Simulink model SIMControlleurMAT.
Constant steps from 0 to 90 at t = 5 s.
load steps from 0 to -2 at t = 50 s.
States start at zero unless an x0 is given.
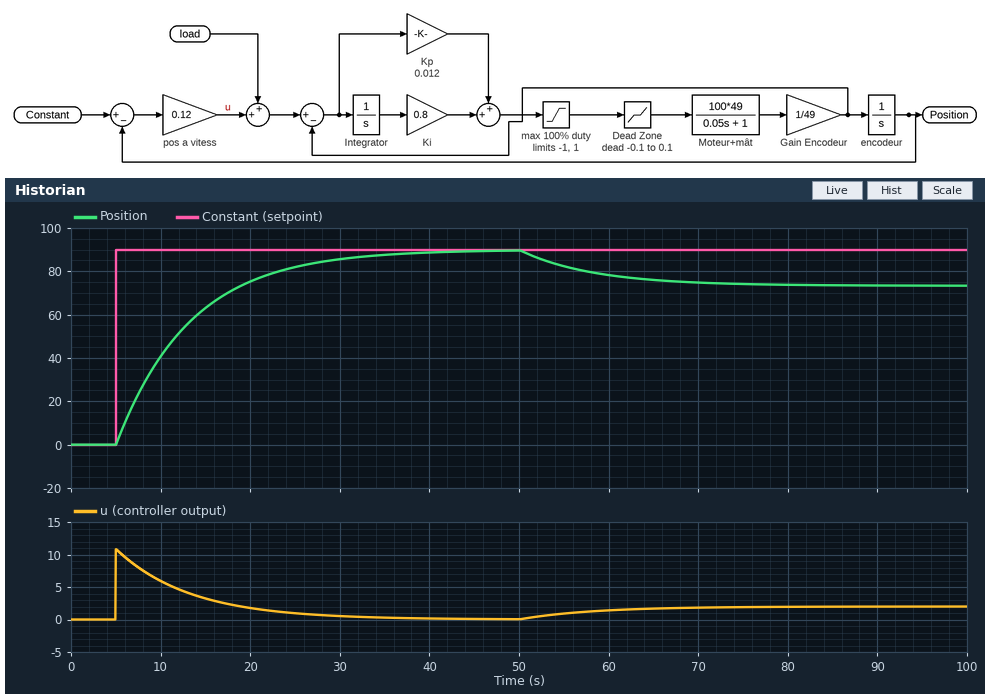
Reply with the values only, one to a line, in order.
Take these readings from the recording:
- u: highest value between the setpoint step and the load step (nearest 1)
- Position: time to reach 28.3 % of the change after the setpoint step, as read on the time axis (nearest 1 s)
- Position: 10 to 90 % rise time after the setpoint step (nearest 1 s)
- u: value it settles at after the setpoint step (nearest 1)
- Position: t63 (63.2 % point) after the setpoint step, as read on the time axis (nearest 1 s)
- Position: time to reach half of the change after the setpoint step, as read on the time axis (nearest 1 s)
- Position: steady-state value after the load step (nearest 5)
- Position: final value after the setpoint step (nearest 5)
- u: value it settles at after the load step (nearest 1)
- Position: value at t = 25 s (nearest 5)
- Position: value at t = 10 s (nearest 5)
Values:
11
8 s
18 s
0
13 s
11 s
75
90
2
80
40
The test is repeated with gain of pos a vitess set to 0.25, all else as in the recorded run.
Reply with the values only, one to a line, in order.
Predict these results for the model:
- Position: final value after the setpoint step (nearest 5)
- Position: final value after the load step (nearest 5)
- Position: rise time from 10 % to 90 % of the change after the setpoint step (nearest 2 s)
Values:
90
80
8 s
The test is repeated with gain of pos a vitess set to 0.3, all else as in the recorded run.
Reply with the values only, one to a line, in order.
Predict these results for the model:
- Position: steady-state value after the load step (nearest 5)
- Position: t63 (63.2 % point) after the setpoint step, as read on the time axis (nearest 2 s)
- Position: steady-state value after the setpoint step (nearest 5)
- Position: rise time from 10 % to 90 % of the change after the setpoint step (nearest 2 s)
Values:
85
8 s
90
8 s
